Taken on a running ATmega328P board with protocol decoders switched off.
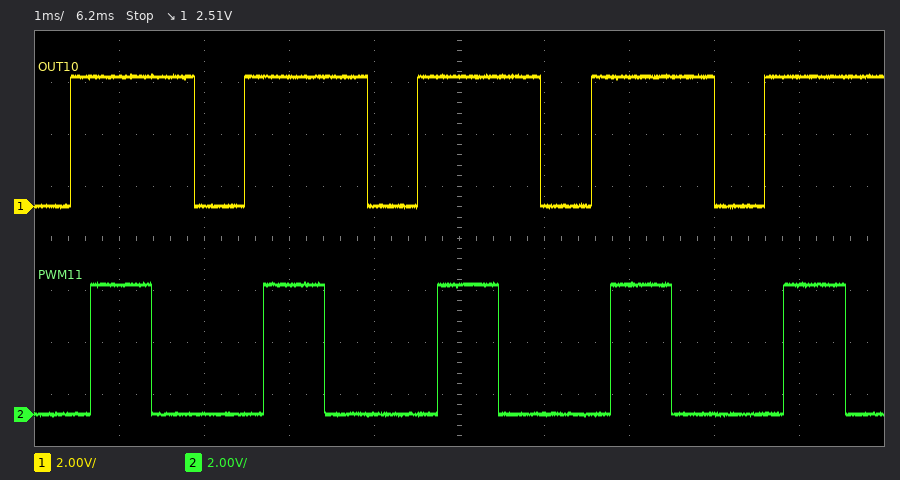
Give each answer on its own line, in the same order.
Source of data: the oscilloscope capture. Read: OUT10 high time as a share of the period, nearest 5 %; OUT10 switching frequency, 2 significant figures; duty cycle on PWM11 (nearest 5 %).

70 %
490 Hz
35 %
